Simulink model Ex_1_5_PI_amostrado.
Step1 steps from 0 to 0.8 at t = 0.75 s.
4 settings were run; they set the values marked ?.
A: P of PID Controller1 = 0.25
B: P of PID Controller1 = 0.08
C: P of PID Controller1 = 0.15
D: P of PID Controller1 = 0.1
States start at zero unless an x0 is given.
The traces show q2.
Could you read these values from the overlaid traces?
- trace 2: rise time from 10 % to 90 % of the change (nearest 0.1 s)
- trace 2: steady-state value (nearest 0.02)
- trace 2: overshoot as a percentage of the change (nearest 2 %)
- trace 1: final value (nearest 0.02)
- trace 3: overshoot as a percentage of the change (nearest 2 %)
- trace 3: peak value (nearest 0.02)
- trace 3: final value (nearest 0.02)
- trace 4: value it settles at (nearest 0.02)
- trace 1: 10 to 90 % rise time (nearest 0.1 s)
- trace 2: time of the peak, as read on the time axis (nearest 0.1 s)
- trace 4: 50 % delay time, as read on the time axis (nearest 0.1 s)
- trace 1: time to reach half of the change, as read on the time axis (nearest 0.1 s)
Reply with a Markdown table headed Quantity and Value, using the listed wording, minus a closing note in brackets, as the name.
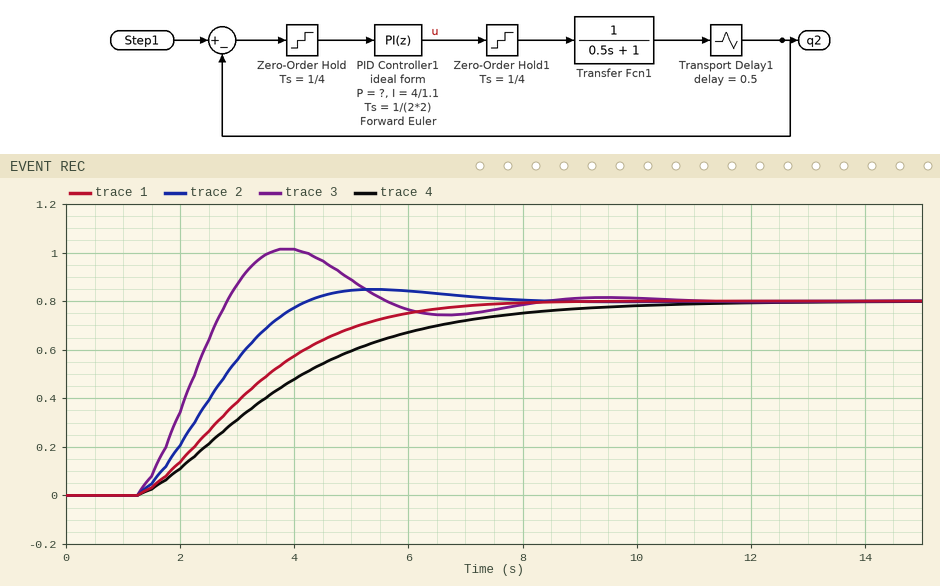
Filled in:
| Quantity | Value |
|---|---|
| trace 2: rise time from 10 % to 90 % of the change | 2.1 s |
| trace 2: steady-state value | 0.80 |
| trace 2: overshoot as a percentage of the change | 6 % |
| trace 1: final value | 0.80 |
| trace 3: overshoot as a percentage of the change | 26 % |
| trace 3: peak value | 1.02 |
| trace 3: final value | 0.80 |
| trace 4: value it settles at | 0.80 |
| trace 1: 10 to 90 % rise time | 3.7 s |
| trace 2: time of the peak, as read on the time axis | 5.5 s |
| trace 4: 50 % delay time, as read on the time axis | 3.5 s |
| trace 1: time to reach half of the change, as read on the time axis | 3.1 s |
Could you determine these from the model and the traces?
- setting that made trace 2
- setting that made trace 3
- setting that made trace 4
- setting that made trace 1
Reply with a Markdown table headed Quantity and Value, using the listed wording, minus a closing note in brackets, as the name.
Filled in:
| Quantity | Value |
|---|---|
| setting that made trace 2 | C |
| setting that made trace 3 | A |
| setting that made trace 4 | B |
| setting that made trace 1 | D |
